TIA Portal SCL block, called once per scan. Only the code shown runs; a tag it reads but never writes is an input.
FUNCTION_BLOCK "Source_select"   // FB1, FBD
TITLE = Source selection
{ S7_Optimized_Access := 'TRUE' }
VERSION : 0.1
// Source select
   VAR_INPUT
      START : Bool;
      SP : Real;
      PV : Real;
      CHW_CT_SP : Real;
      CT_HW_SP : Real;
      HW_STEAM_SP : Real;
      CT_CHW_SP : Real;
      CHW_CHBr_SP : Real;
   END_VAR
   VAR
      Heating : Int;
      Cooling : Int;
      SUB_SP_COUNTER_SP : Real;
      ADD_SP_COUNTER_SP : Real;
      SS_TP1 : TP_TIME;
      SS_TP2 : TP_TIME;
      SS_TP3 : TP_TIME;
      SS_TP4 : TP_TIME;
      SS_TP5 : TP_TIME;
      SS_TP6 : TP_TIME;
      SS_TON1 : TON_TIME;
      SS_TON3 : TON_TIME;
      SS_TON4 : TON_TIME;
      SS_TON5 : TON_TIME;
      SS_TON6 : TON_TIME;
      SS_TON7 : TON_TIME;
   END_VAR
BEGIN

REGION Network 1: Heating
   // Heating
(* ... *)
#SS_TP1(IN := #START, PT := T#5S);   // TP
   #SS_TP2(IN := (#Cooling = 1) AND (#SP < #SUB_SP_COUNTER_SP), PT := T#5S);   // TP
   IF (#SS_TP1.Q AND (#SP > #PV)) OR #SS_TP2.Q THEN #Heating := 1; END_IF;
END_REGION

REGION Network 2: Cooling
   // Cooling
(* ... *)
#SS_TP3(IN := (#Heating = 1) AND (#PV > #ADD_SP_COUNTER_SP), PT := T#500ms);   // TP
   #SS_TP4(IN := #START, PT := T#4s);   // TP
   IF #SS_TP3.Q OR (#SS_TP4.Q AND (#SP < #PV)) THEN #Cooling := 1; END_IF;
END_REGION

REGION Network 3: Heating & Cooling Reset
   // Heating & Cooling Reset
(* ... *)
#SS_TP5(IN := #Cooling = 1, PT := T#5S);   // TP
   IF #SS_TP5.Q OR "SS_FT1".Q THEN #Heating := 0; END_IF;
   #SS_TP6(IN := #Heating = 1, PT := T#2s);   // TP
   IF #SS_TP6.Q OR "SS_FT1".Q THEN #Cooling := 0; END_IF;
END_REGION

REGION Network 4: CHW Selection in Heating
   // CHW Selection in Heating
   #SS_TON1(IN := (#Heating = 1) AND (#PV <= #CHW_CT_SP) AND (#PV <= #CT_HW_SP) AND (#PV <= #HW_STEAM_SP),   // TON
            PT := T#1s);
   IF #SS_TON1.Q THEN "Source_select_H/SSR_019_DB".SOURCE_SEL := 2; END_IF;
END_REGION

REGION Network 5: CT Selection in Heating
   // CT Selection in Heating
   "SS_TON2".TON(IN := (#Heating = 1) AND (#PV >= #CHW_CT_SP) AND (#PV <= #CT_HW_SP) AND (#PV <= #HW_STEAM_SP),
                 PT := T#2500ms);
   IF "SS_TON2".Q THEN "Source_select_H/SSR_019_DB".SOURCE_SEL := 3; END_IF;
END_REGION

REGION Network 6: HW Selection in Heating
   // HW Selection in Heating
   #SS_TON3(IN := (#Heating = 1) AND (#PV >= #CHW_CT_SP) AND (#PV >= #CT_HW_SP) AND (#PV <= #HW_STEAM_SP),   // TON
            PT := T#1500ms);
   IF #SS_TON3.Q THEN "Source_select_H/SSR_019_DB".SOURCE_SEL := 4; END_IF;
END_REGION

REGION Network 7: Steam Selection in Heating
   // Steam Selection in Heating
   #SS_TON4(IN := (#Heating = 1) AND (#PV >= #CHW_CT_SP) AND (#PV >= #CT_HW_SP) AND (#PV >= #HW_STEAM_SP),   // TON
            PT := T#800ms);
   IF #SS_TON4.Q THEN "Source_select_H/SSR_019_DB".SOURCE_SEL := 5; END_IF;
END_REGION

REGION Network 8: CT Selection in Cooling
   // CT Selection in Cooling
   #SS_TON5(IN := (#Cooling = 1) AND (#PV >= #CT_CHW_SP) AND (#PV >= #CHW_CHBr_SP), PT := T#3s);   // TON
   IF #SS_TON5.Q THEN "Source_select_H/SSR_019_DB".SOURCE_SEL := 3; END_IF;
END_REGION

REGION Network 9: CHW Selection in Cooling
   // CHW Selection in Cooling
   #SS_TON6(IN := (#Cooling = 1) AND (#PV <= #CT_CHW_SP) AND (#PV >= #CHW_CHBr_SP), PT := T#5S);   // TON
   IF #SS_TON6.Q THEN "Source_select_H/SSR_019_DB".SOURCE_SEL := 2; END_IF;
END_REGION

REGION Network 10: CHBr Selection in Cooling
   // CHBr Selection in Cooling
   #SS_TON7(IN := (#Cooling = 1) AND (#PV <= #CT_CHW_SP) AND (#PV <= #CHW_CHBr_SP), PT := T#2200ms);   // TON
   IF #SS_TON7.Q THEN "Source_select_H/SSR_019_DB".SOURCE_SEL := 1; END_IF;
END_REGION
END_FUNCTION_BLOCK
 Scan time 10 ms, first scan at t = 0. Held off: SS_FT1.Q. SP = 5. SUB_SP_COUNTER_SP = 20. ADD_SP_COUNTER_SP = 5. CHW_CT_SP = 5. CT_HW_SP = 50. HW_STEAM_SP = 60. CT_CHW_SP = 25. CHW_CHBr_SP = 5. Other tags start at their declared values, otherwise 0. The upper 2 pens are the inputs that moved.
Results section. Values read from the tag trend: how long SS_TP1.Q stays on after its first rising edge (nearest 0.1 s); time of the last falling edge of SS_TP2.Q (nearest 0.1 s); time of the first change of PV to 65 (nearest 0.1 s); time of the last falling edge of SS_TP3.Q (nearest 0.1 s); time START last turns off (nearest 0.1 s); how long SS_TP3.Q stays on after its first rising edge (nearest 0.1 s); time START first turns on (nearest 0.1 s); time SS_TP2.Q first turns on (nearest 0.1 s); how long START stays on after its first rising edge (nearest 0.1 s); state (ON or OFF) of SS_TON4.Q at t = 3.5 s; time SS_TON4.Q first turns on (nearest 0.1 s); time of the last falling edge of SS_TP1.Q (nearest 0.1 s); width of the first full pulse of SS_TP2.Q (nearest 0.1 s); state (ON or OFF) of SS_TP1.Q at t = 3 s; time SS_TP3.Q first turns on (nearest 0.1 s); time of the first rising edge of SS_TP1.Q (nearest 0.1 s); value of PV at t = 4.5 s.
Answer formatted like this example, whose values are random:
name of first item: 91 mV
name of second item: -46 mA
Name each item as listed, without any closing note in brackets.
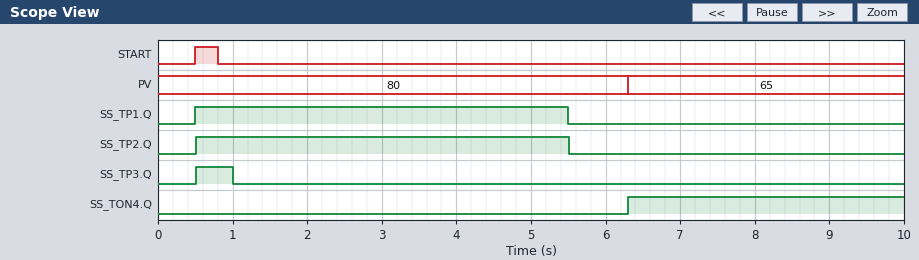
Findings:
how long SS_TP1.Q stays on after its first rising edge: 5.0 s
time of the last falling edge of SS_TP2.Q: 5.5 s
time of the first change of PV to 65: 6.3 s
time of the last falling edge of SS_TP3.Q: 1.0 s
time START last turns off: 0.8 s
how long SS_TP3.Q stays on after its first rising edge: 0.5 s
time START first turns on: 0.5 s
time SS_TP2.Q first turns on: 0.5 s
how long START stays on after its first rising edge: 0.3 s
state (ON or OFF) of SS_TON4.Q at t = 3.5 s: OFF
time SS_TON4.Q first turns on: 6.3 s
time of the last falling edge of SS_TP1.Q: 5.5 s
width of the first full pulse of SS_TP2.Q: 5.0 s
state (ON or OFF) of SS_TP1.Q at t = 3 s: ON
time SS_TP3.Q first turns on: 0.5 s
time of the first rising edge of SS_TP1.Q: 0.5 s
value of PV at t = 4.5 s: 80
